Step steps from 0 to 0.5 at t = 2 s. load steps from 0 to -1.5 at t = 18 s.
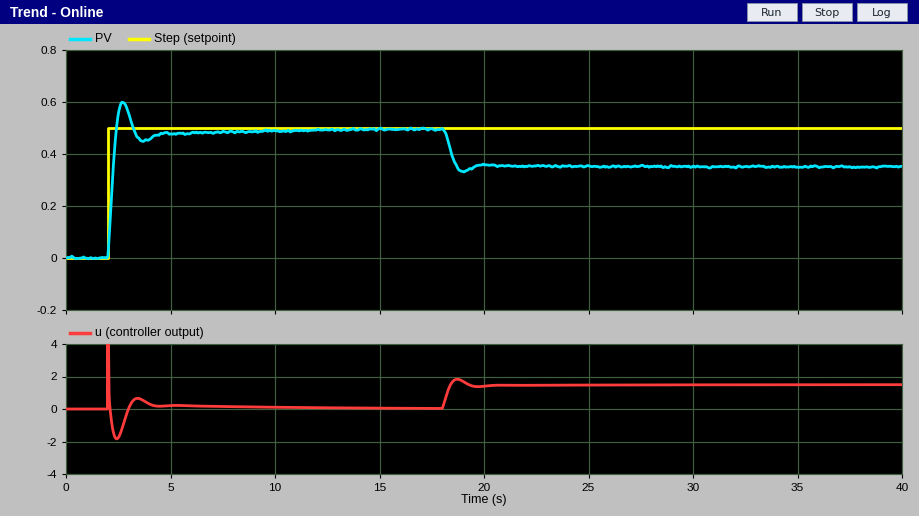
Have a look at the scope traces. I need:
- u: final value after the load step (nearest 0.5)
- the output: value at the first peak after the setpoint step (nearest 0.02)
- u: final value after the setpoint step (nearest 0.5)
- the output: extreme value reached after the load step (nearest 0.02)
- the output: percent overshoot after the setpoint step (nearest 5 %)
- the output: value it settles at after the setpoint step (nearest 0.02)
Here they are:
1.5
0.60
0.0
0.34
20 %
0.50
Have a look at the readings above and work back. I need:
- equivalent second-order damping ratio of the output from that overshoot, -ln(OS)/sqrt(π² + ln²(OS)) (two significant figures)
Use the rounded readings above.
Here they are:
0.46
